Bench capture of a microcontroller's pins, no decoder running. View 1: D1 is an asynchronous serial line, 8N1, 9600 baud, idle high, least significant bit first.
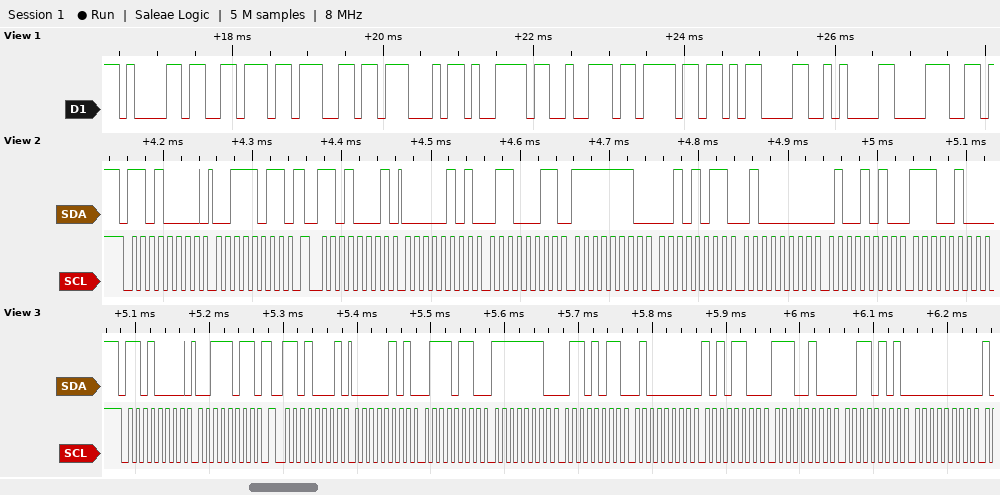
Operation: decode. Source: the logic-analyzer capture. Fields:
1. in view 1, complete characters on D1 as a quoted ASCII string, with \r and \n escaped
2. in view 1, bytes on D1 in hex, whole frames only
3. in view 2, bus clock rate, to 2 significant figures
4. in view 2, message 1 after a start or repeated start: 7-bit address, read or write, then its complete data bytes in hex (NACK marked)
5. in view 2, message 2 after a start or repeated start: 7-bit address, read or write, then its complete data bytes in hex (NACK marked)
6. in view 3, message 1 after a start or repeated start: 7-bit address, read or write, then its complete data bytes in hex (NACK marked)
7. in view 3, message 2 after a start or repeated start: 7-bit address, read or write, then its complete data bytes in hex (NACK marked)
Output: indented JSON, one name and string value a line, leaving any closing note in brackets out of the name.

{
  "in view 1, complete characters on D1 as a quoted ASCII string, with \\r and \\n escaped": "\"avgGyro\\r\\n8\"",
  "in view 1, bytes on D1 in hex, whole frames only": "61 76 67 47 79 72 6F 0D 0A 38",
  "in view 2, bus clock rate, to 2 significant figures": "100 kHz",
  "in view 2, message 1 after a start or repeated start: 7-bit address, read or write, then its complete data bytes in hex": "0x68 write: 3B",
  "in view 2, message 2 after a start or repeated start: 7-bit address, read or write, then its complete data bytes in hex": "0x68 read: 05 63 FE 2B 40 4A E4",
  "in view 3, message 1 after a start or repeated start: 7-bit address, read or write, then its complete data bytes in hex": "0x68 write: 3B",
  "in view 3, message 2 after a start or repeated start: 7-bit address, read or write, then its complete data bytes in hex": "0x68 read: 05 76 FE 6B 40 AC E4 35 00"
}
